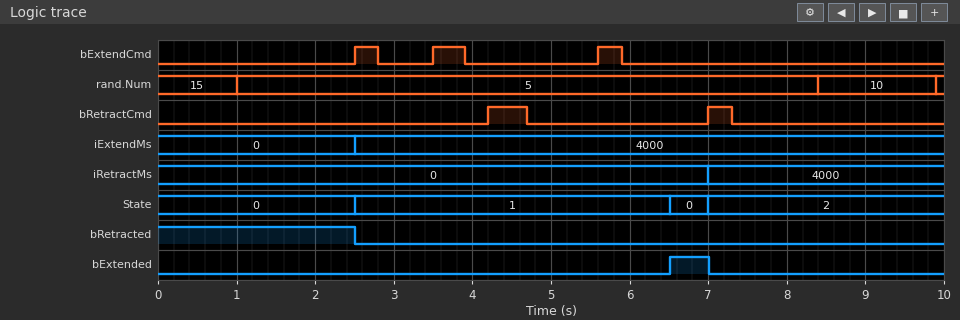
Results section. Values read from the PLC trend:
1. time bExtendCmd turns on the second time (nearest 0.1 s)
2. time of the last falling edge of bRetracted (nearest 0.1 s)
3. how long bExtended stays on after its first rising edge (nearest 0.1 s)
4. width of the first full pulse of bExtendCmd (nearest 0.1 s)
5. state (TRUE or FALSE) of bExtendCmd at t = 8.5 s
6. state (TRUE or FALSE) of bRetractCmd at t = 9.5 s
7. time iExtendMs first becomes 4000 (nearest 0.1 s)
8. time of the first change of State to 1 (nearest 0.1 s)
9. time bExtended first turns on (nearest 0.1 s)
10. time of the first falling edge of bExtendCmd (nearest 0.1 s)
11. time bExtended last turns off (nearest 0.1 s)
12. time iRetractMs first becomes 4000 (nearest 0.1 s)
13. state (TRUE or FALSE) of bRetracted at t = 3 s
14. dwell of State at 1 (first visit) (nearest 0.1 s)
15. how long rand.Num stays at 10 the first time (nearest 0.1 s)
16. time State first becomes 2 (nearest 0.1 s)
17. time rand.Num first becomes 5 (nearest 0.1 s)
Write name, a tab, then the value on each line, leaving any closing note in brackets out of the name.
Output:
time bExtendCmd turns on the second time	3.5 s
time of the last falling edge of bRetracted	2.5 s
how long bExtended stays on after its first rising edge	0.5 s
width of the first full pulse of bExtendCmd	0.3 s
state (TRUE or FALSE) of bExtendCmd at t = 8.5 s	FALSE
state (TRUE or FALSE) of bRetractCmd at t = 9.5 s	FALSE
time iExtendMs first becomes 4000	2.5 s
time of the first change of State to 1	2.5 s
time bExtended first turns on	6.5 s
time of the first falling edge of bExtendCmd	2.8 s
time bExtended last turns off	7.0 s
time iRetractMs first becomes 4000	7.0 s
state (TRUE or FALSE) of bRetracted at t = 3 s	FALSE
dwell of State at 1 (first visit)	4.0 s
how long rand.Num stays at 10 the first time	1.5 s
time State first becomes 2	7.0 s
time rand.Num first becomes 5	1.0 s
